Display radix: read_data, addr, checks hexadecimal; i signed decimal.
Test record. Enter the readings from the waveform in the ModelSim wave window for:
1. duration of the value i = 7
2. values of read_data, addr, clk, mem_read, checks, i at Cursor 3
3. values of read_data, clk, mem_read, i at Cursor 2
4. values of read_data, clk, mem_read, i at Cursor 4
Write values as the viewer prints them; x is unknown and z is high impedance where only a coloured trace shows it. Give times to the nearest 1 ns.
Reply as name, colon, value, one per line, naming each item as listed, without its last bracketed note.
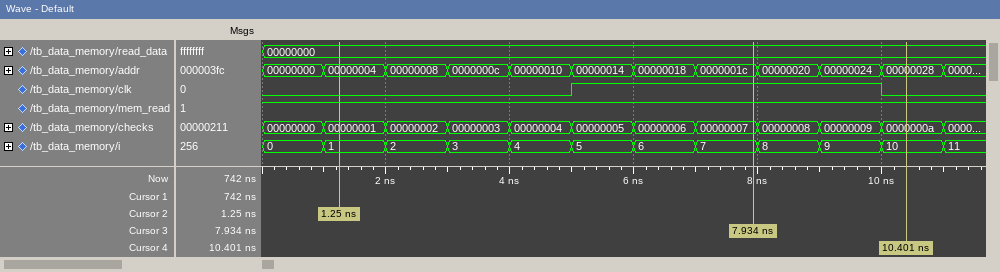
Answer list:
duration of the value i = 7: 1 ns
values of read_data, addr, clk, mem_read, checks, i at Cursor 3: read_data=00000000, addr=0000001c, clk=1, mem_read=1, checks=00000007, i=7
values of read_data, clk, mem_read, i at Cursor 2: read_data=00000000, clk=0, mem_read=1, i=1
values of read_data, clk, mem_read, i at Cursor 4: read_data=00000000, clk=0, mem_read=1, i=10
